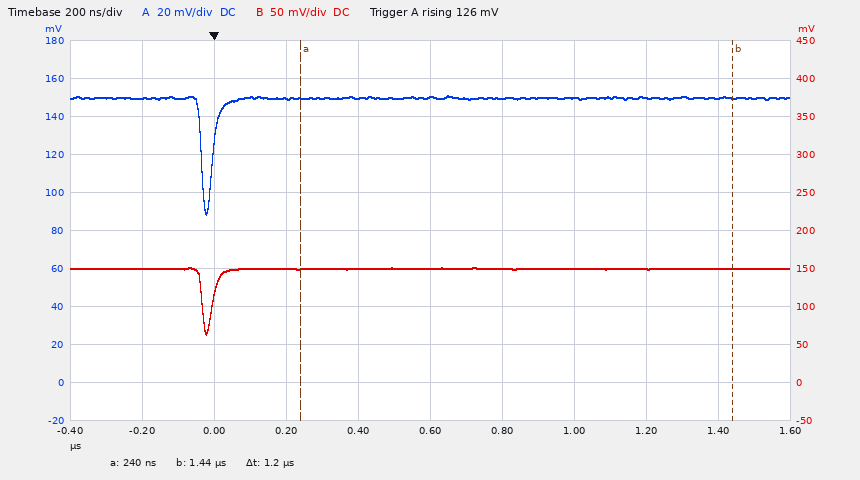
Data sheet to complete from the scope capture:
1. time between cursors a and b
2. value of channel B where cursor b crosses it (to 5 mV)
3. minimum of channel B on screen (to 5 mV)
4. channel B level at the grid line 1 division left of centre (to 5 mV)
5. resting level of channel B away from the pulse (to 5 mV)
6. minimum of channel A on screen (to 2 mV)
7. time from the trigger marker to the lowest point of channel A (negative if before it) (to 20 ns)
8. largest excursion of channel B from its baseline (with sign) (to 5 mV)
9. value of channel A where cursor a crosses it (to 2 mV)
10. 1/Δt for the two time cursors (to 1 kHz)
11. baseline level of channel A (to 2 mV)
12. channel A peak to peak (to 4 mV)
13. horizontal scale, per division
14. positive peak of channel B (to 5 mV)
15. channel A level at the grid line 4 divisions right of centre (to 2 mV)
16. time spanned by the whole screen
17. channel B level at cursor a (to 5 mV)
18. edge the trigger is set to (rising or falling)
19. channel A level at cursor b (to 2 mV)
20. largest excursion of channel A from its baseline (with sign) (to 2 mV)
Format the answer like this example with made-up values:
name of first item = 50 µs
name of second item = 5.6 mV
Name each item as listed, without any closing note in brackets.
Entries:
time between cursors a and b = 1.2 µs
value of channel B where cursor b crosses it = 150 mV
minimum of channel B on screen = 65 mV
channel B level at the grid line 1 division left of centre = 150 mV
resting level of channel B away from the pulse = 150 mV
minimum of channel A on screen = 88 mV
time from the trigger marker to the lowest point of channel A (negative if before it) = -20 ns
largest excursion of channel B from its baseline (with sign) = -85 mV
value of channel A where cursor a crosses it = 150 mV
1/Δt for the two time cursors = 833 kHz
baseline level of channel A = 150 mV
channel A peak to peak = 64 mV
horizontal scale, per division = 200 ns
positive peak of channel B = 150 mV
channel A level at the grid line 4 divisions right of centre = 150 mV
time spanned by the whole screen = 2 µs
channel B level at cursor a = 150 mV
edge the trigger is set to = rising
channel A level at cursor b = 150 mV
largest excursion of channel A from its baseline (with sign) = -62 mV
